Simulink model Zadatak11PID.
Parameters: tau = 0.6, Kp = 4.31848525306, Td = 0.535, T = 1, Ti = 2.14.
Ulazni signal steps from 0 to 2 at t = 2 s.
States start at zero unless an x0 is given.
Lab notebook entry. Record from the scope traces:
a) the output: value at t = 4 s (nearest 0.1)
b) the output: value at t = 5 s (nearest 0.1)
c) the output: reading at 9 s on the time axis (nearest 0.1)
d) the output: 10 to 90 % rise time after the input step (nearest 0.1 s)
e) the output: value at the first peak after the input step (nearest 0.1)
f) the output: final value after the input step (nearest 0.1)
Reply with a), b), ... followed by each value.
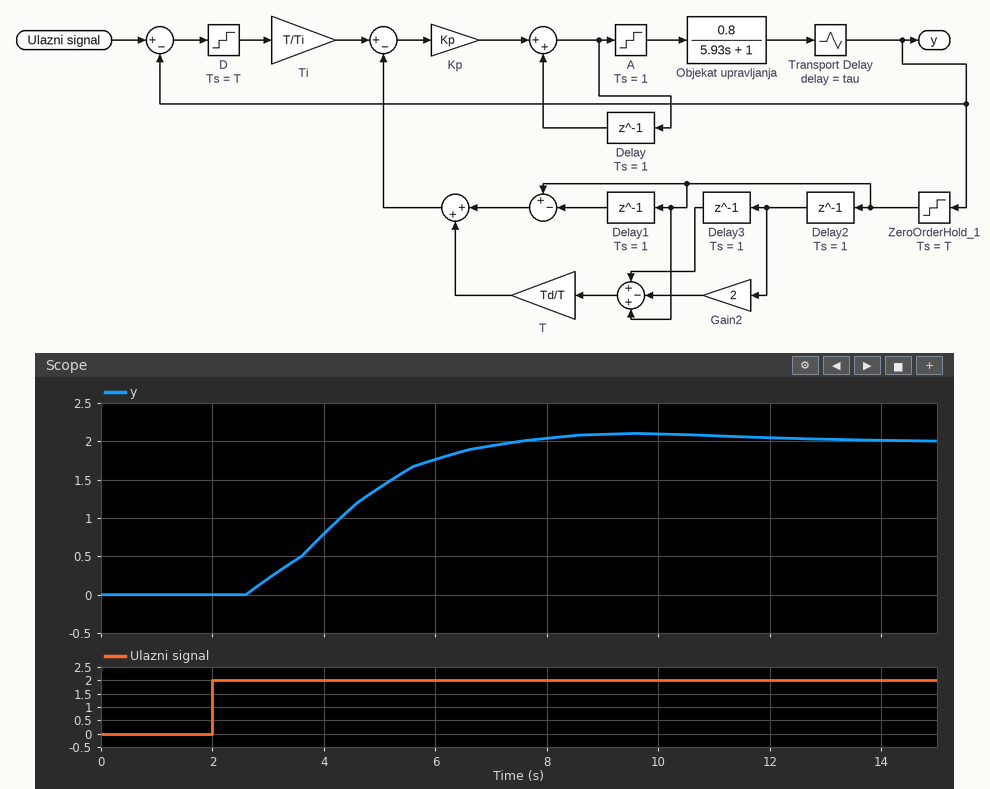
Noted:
a) 0.8
b) 1.4
c) 2.1
d) 3.2 s
e) 2.1
f) 2.0
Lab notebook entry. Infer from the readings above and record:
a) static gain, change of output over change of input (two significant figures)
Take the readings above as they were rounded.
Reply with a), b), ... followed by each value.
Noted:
a) 1.0
